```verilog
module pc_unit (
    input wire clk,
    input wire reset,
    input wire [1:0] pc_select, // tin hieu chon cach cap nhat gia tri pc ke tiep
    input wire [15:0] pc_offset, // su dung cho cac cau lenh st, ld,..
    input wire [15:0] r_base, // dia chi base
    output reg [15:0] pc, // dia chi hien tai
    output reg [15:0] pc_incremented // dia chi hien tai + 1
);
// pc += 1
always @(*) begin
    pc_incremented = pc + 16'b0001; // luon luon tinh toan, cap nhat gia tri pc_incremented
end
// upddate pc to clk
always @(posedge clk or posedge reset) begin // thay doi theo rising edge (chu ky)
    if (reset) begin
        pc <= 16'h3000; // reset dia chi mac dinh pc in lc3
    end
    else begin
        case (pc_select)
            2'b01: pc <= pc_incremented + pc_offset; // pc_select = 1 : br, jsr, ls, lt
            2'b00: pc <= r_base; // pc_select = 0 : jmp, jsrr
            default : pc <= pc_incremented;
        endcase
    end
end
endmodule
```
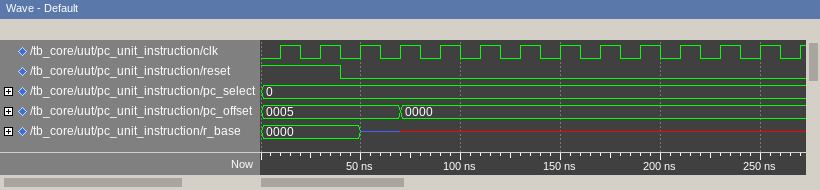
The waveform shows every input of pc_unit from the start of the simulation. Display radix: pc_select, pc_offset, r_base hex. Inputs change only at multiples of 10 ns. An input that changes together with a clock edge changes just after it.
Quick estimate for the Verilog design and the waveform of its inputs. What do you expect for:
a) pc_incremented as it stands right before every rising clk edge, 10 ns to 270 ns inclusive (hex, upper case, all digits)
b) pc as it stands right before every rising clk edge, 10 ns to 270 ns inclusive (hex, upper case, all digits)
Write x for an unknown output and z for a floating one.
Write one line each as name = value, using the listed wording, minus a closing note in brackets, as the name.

pc_incremented as it stands right before every rising clk edge, 10 ns to 270 ns inclusive = 3001, 3001, 3001, 0001, x, x, x, x, x, x, x, x, x, x
pc as it stands right before every rising clk edge, 10 ns to 270 ns inclusive = 3000, 3000, 3000, 0000, z, x, x, x, x, x, x, x, x, x
